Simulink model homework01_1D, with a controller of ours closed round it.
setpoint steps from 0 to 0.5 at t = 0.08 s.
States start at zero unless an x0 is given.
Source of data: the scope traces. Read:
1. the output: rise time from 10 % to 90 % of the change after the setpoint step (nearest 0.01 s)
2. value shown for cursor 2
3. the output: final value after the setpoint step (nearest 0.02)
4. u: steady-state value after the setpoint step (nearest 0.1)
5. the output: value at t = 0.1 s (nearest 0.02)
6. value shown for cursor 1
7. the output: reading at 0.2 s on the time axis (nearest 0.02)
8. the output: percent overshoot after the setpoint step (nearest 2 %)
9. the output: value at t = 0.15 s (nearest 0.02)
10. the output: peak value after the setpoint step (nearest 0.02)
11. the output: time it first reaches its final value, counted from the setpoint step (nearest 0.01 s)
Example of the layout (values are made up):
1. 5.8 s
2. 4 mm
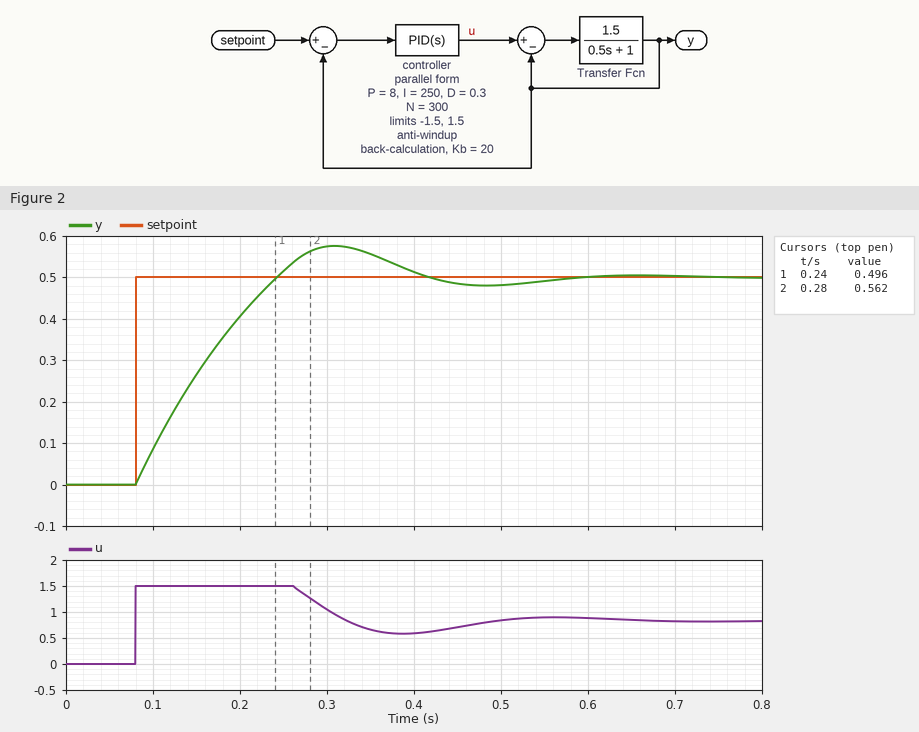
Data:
1. 0.13 s
2. 0.562
3. 0.50
4. 0.8
5. 0.08
6. 0.496
7. 0.40
8. 16 %
9. 0.26
10. 0.58
11. 0.16 s
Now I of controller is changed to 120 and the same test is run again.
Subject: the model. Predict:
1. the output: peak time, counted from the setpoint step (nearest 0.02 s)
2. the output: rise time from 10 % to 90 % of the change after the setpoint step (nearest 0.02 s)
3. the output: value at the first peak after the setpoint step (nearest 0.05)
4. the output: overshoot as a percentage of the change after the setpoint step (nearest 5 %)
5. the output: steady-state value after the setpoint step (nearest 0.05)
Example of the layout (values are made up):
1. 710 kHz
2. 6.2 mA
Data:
1. 0.26 s
2. 0.14 s
3. 0.55
4. 10 %
5. 0.50
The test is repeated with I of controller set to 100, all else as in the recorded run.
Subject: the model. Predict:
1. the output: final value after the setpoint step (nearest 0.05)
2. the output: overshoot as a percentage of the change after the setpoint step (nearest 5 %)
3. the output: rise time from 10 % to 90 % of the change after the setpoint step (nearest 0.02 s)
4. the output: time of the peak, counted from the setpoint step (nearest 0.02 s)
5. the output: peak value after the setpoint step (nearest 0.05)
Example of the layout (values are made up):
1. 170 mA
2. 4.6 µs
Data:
1. 0.50
2. 10 %
3. 0.16 s
4. 0.30 s
5. 0.55
